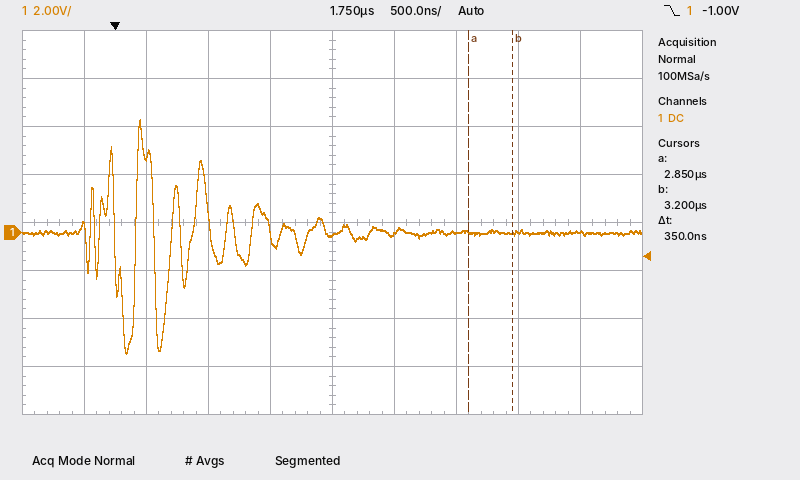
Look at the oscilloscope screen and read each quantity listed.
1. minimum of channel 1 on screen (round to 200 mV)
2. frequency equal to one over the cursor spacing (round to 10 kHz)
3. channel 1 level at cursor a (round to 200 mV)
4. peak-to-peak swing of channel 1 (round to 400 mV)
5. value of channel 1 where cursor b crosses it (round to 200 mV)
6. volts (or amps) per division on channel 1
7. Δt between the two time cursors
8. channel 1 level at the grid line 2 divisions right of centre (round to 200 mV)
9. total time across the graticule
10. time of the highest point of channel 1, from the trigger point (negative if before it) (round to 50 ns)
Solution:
-5.0 V
2.86 MHz
0.0 V
9.6 V
0.0 V
2 V
350 ns
0.0 V
5 µs
+200 ns
